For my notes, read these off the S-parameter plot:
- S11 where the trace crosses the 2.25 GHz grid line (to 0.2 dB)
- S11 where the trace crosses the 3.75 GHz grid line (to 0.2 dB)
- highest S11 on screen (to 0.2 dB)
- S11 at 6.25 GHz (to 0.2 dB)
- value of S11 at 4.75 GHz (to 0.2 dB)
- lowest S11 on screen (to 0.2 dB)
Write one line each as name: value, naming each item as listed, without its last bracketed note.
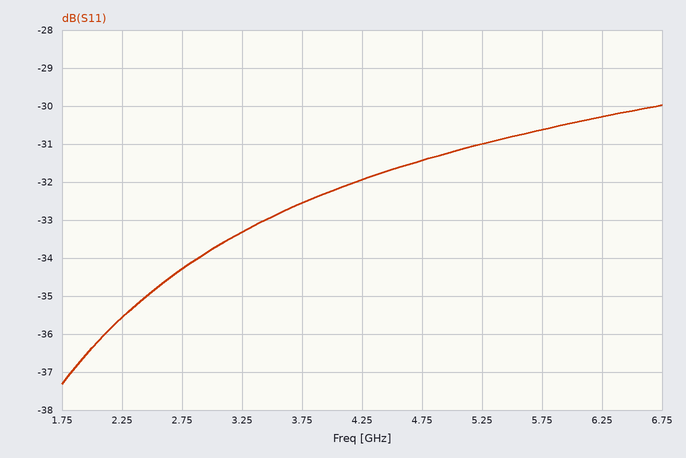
S11 where the trace crosses the 2.25 GHz grid line: -35.6 dB
S11 where the trace crosses the 3.75 GHz grid line: -32.6 dB
highest S11 on screen: -30.0 dB
S11 at 6.25 GHz: -30.2 dB
value of S11 at 4.75 GHz: -31.4 dB
lowest S11 on screen: -37.4 dB
